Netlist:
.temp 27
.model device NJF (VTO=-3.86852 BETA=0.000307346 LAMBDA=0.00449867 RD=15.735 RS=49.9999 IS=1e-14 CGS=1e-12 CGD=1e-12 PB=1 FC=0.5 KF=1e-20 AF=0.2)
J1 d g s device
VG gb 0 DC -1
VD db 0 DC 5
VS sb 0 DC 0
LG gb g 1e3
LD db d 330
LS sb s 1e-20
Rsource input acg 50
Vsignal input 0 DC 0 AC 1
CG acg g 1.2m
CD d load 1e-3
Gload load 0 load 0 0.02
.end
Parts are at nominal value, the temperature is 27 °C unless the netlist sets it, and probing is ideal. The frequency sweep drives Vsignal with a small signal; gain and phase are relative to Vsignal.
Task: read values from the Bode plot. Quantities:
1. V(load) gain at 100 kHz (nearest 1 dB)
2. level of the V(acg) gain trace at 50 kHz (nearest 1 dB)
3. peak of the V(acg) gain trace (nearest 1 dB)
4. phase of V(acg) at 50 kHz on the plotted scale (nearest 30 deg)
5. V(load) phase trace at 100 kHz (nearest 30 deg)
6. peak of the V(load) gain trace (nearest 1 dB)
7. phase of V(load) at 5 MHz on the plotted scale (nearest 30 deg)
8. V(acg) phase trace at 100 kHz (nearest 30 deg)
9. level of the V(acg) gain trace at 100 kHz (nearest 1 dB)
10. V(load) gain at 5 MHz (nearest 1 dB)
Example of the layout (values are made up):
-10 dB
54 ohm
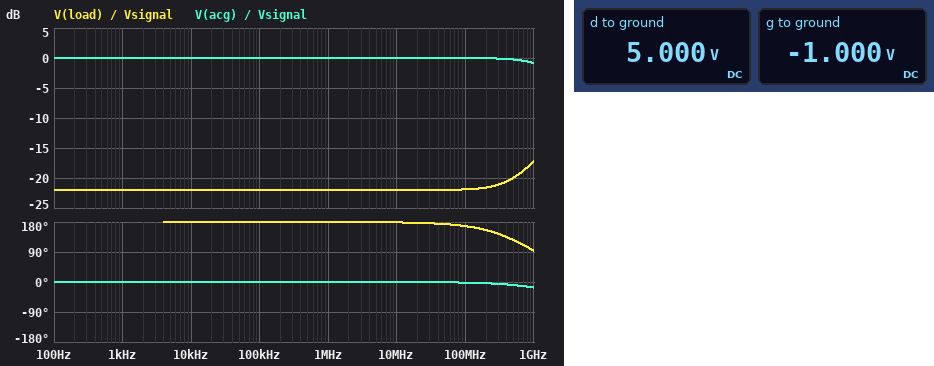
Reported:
-22 dB
0 dB
0 dB
0 deg
180 deg
-17 dB
180 deg
0 deg
0 dB
-22 dB
